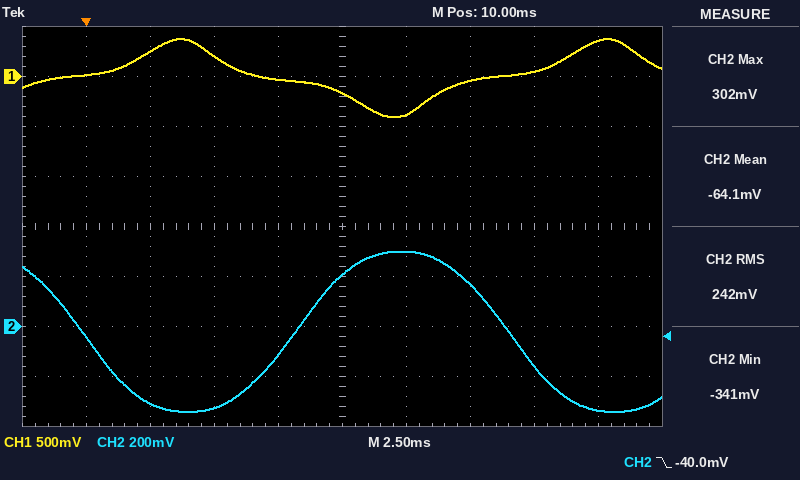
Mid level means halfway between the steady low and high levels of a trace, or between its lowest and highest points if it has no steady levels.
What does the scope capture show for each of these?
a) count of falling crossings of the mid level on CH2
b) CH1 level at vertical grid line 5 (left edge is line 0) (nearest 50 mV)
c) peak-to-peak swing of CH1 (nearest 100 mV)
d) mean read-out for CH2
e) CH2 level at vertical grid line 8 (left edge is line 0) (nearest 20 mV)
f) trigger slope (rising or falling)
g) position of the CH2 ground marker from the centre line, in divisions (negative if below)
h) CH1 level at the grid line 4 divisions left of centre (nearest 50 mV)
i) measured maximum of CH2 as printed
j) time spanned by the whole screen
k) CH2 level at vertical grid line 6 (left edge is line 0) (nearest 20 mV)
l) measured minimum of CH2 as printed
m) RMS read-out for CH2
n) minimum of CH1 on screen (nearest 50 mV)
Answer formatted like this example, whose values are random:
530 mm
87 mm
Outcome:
2
-150 mV
800 mV
-64.1 mV
-160 mV
falling
-2.0 div
0 mV
302 mV
25 ms
300 mV
-341 mV
242 mV
-400 mV
